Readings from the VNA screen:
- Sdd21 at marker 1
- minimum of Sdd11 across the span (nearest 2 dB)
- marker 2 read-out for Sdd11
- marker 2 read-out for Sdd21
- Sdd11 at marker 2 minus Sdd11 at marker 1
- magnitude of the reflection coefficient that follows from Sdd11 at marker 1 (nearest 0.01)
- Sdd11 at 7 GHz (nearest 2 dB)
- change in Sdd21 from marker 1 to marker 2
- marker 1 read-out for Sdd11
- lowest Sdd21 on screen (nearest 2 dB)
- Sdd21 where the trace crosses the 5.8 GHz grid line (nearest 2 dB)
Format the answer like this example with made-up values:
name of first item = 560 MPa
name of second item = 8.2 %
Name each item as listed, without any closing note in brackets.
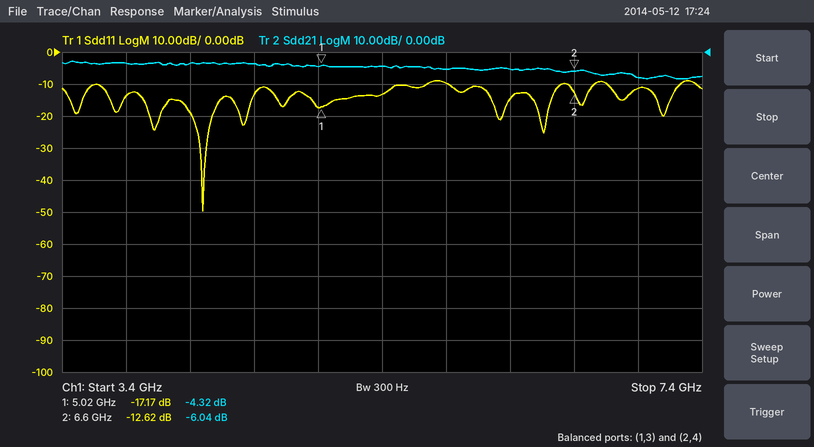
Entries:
Sdd21 at marker 1 = -4.32 dB
minimum of Sdd11 across the span = -50 dB
marker 2 read-out for Sdd11 = -12.62 dB
marker 2 read-out for Sdd21 = -6.04 dB
Sdd11 at marker 2 minus Sdd11 at marker 1 = 4.55 dB
magnitude of the reflection coefficient that follows from Sdd11 at marker 1 = 0.14
Sdd11 at 7 GHz = -12 dB
change in Sdd21 from marker 1 to marker 2 = -1.72 dB
marker 1 read-out for Sdd11 = -17.17 dB
lowest Sdd21 on screen = -8 dB
Sdd21 where the trace crosses the 5.8 GHz grid line = -6 dB
